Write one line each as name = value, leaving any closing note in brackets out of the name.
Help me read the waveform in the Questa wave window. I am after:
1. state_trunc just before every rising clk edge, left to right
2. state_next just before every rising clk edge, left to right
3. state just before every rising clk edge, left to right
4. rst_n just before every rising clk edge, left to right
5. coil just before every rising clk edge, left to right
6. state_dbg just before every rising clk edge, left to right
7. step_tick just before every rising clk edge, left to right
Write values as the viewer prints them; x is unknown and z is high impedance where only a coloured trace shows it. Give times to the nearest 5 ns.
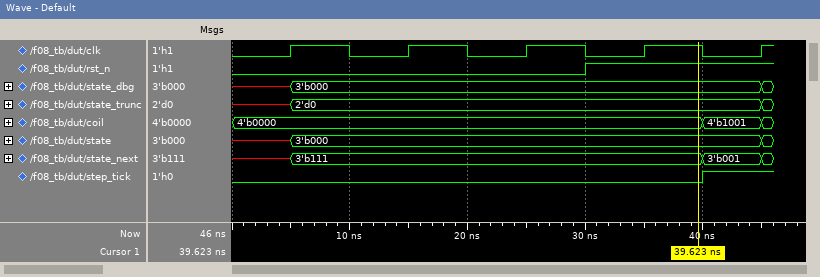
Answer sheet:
state_trunc just before every rising clk edge, left to right = x, 2'd0, 2'd0, 2'd0, 2'd0
state_next just before every rising clk edge, left to right = x, 3'b111, 3'b111, 3'b111, 3'b001
state just before every rising clk edge, left to right = x, 3'b000, 3'b000, 3'b000, 3'b000
rst_n just before every rising clk edge, left to right = 0 0 0 1 1
coil just before every rising clk edge, left to right = 4'b0000, 4'b0000, 4'b0000, 4'b0000, 4'b1001
state_dbg just before every rising clk edge, left to right = x, 3'b000, 3'b000, 3'b000, 3'b000
step_tick just before every rising clk edge, left to right = 0 0 0 0 1
